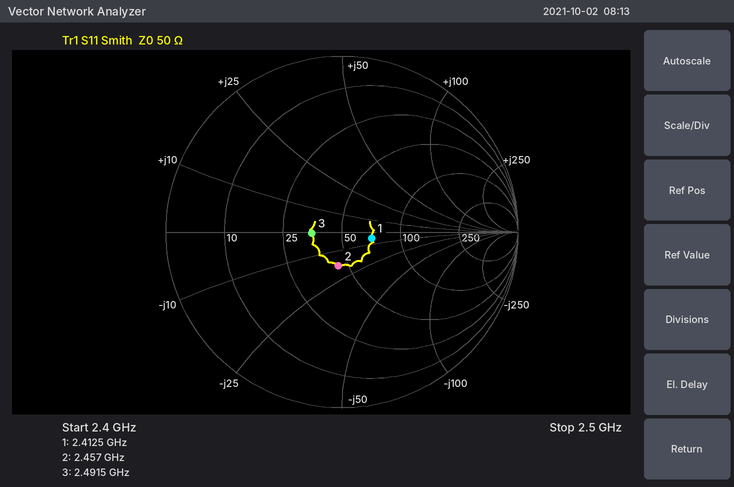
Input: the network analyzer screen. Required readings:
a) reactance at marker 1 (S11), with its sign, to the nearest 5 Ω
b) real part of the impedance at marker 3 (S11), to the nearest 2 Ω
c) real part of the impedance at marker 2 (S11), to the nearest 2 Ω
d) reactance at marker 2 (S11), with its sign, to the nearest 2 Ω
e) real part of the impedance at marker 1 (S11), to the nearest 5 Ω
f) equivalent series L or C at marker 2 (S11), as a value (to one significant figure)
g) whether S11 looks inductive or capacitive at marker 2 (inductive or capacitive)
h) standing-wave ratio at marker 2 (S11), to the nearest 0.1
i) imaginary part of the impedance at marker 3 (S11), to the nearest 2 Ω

-5 Ω
36 Ω
44 Ω
-18 Ω
70 Ω
4 pF
capacitive
1.5
0 Ω
